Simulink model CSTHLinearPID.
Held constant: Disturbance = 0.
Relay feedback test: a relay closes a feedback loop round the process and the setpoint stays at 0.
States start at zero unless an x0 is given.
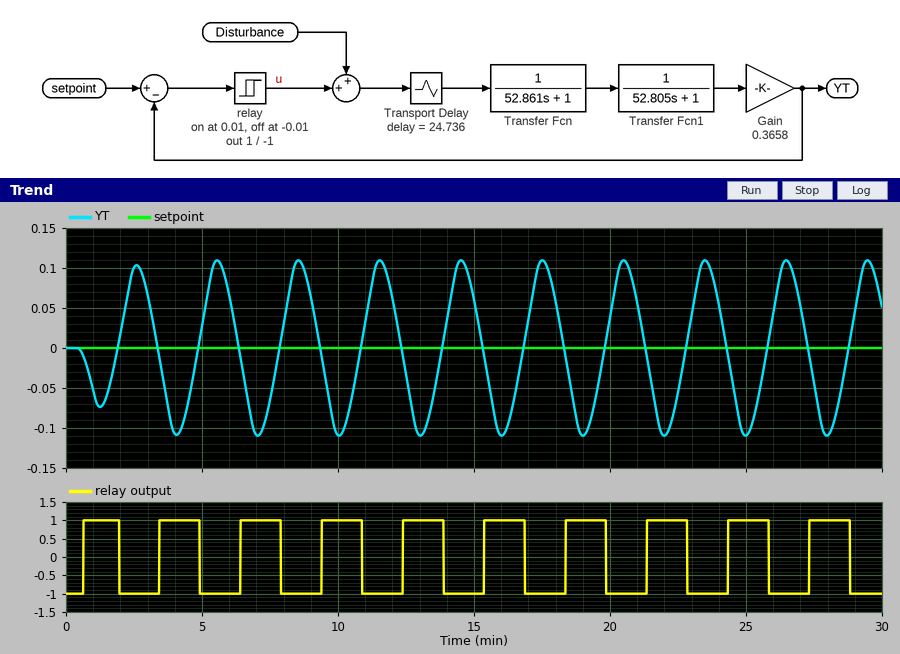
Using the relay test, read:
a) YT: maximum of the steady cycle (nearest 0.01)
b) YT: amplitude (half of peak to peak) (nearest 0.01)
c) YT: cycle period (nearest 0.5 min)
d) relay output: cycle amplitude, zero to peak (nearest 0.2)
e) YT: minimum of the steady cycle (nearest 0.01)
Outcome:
0.11
0.11
3.0 min
1.0
-0.11
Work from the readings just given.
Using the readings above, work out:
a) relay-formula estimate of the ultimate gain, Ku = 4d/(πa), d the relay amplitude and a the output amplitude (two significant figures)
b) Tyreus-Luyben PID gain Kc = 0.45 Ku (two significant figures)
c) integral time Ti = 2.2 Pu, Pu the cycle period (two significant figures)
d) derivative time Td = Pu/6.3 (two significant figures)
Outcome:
12
5.4
6.6 min
0.48 min
